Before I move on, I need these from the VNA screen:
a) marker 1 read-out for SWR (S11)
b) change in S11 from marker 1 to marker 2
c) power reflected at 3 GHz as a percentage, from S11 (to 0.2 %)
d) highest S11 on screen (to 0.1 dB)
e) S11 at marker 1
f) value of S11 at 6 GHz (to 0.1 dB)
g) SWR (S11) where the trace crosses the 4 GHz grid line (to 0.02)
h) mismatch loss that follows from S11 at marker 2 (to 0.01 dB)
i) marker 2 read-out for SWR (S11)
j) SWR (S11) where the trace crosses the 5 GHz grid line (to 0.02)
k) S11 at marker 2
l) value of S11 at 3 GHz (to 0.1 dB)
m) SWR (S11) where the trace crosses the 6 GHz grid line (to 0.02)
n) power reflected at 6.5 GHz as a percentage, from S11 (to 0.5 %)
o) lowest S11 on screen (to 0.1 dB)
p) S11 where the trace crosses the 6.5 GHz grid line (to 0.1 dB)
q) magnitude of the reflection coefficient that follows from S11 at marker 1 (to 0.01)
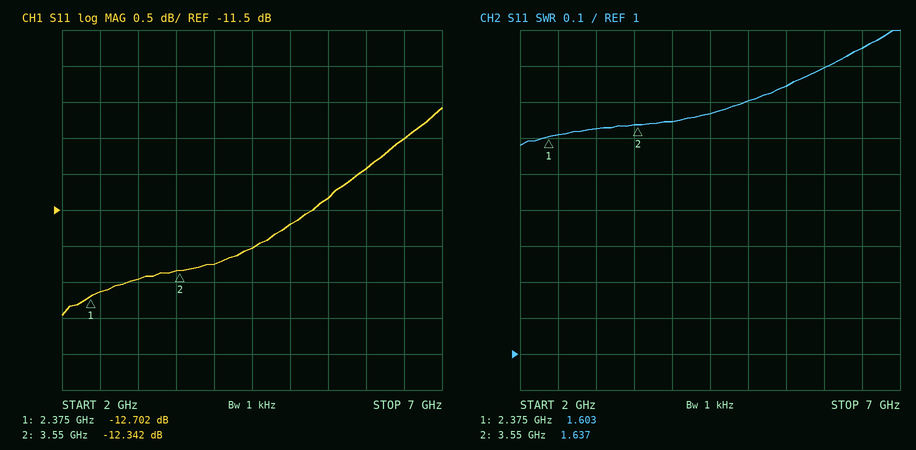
1.603
0.360 dB
5.6 %
-10.1 dB
-12.702 dB
-10.9 dB
1.64
0.26 dB
1.637
1.70
-12.342 dB
-12.5 dB
1.80
9.0 %
-13.0 dB
-10.5 dB
0.23
